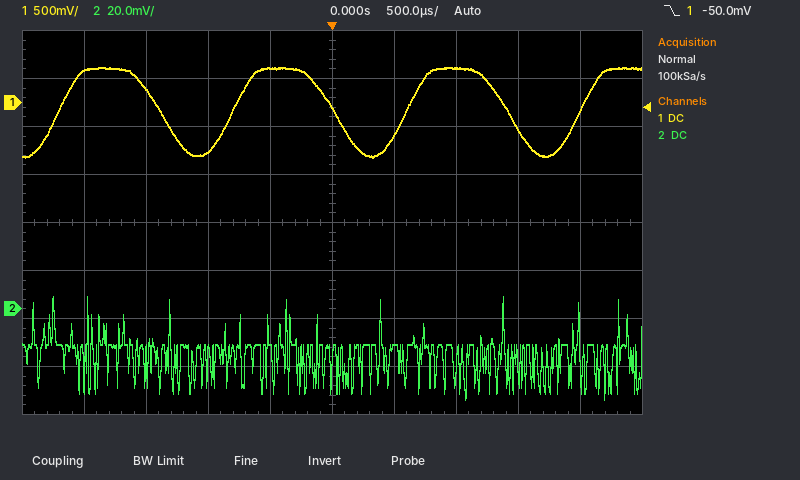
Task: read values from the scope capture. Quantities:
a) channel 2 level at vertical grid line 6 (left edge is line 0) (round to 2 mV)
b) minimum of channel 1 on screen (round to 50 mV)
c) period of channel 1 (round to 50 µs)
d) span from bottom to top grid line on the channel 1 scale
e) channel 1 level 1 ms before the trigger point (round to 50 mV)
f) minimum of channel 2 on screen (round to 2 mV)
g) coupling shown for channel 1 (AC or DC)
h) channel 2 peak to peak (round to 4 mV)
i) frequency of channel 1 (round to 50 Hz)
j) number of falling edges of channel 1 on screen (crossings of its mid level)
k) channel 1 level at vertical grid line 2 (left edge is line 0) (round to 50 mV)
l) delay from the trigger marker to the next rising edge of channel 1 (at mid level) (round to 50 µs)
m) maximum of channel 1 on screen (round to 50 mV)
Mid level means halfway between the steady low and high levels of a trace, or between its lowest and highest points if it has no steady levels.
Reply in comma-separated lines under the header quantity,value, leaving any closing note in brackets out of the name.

quantity,value
channel 2 level at vertical grid line 6 (left edge is line 0),-16 mV
minimum of channel 1 on screen,-550 mV
period of channel 1,1.40 ms
span from bottom to top grid line on the channel 1 scale,4 V
channel 1 level 1 ms before the trigger point,-500 mV
minimum of channel 2 on screen,-38 mV
coupling shown for channel 1,DC
channel 2 peak to peak,44 mV
frequency of channel 1,700 Hz
number of falling edges of channel 1 on screen,3
channel 1 level at vertical grid line 2 (left edge is line 0),150 mV
delay from the trigger marker to the next rising edge of channel 1 (at mid level),600 µs
maximum of channel 1 on screen,350 mV
